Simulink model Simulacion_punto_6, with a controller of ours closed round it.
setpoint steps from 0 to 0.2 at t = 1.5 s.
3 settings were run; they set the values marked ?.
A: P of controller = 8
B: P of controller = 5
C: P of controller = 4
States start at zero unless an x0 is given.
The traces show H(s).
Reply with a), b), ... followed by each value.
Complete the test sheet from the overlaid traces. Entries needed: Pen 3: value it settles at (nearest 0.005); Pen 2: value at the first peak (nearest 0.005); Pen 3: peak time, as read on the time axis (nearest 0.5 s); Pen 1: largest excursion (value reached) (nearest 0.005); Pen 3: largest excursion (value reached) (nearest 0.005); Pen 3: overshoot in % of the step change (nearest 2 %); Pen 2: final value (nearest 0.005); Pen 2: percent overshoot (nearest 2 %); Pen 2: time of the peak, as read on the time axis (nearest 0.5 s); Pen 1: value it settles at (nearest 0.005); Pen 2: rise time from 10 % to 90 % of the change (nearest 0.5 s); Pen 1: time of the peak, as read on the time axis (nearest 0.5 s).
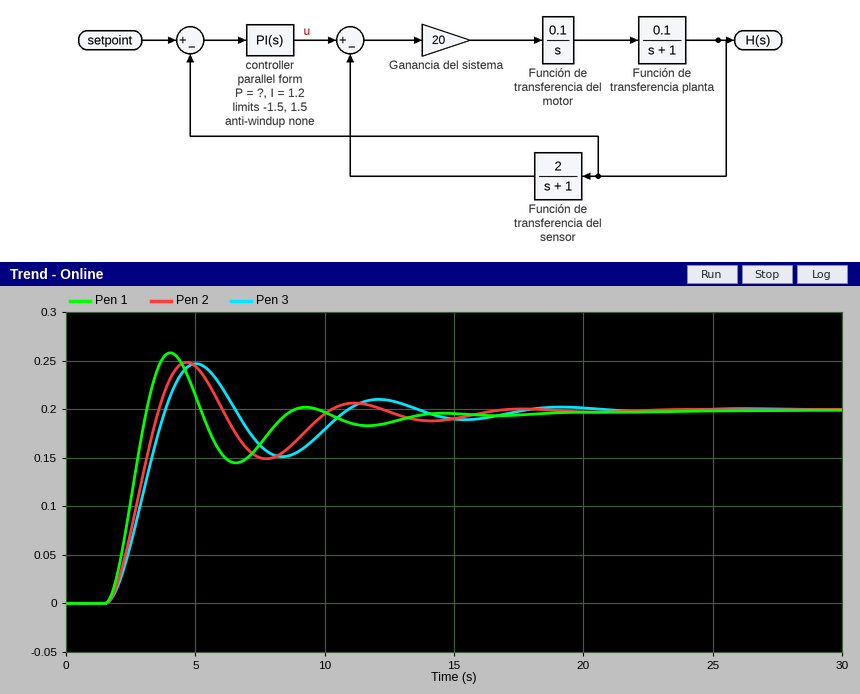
a) 0.200
b) 0.250
c) 5.0 s
d) 0.260
e) 0.245
f) 24 %
g) 0.200
h) 24 %
i) 4.5 s
j) 0.200
k) 1.5 s
l) 4.0 s
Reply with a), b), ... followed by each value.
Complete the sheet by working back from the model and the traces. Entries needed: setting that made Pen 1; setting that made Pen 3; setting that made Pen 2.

a) A
b) C
c) B
